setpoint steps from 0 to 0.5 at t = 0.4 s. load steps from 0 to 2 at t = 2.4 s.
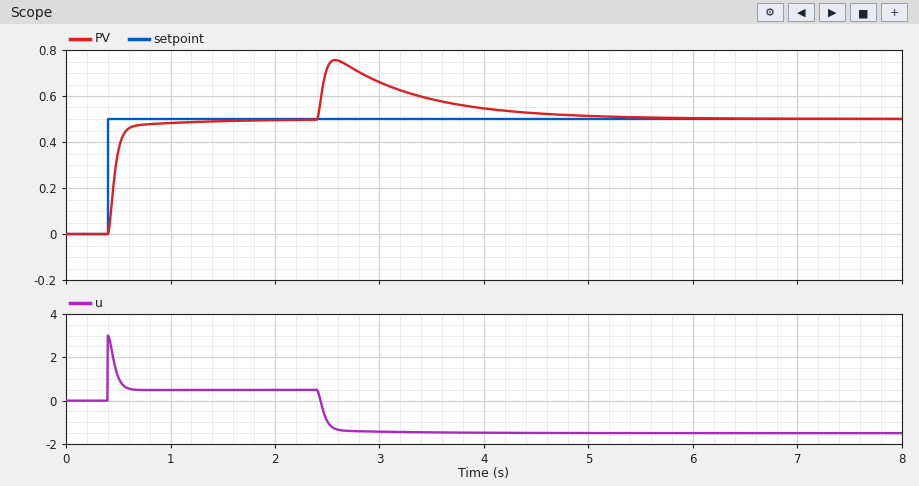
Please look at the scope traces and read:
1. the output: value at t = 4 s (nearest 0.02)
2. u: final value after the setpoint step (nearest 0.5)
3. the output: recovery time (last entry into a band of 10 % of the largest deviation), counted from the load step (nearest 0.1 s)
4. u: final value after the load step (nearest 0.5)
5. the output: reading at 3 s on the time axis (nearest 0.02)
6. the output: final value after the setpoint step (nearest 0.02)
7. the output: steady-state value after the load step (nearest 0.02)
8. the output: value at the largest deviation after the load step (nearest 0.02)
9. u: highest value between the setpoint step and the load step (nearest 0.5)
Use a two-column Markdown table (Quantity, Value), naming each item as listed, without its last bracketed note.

| Quantity | Value |
|---|---|
| the output: value at t = 4 s | 0.54 |
| u: final value after the setpoint step | 0.5 |
| the output: recovery time (last entry into a band of 10 % of the largest deviation), counted from the load step | 2.1 s |
| u: final value after the load step | -1.5 |
| the output: reading at 3 s on the time axis | 0.66 |
| the output: final value after the setpoint step | 0.50 |
| the output: steady-state value after the load step | 0.50 |
| the output: value at the largest deviation after the load step | 0.76 |
| u: highest value between the setpoint step and the load step | 3.0 |
